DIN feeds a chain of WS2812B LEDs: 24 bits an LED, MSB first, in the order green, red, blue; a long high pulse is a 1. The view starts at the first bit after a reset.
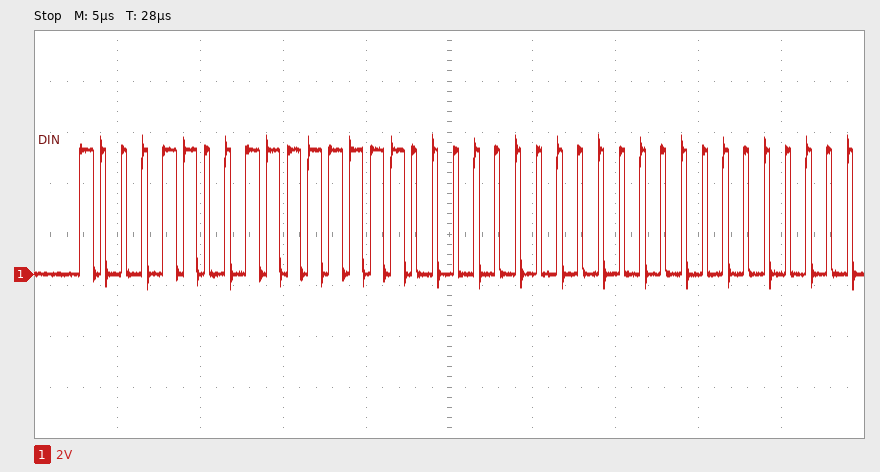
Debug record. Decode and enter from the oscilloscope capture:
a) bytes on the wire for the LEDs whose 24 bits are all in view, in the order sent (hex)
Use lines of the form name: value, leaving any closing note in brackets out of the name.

bytes on the wire for the LEDs whose 24 bits are all in view, in the order sent: 8C FF 00
